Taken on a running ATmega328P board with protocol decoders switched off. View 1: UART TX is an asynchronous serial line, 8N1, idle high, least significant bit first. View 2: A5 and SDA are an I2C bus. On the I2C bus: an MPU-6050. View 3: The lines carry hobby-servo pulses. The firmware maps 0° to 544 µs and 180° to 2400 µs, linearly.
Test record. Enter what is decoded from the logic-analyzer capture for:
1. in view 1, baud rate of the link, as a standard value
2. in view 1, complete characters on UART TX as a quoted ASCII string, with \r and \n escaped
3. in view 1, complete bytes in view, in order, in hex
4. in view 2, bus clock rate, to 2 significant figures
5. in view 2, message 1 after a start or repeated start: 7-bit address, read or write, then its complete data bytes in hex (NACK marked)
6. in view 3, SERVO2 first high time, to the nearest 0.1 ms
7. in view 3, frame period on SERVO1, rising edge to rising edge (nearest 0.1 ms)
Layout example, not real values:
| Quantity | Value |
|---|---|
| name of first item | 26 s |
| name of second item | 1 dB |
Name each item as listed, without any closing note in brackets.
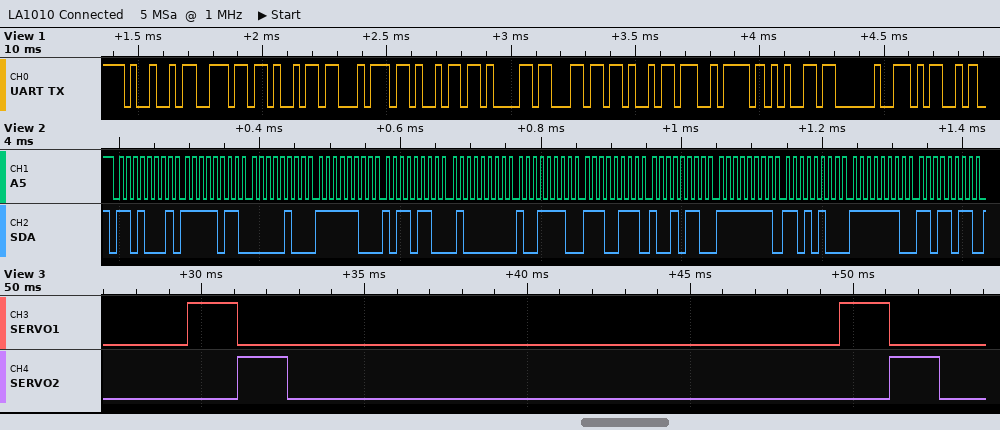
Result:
| Quantity | Value |
|---|---|
| in view 1, baud rate of the link, as a standard value | 38400 baud |
| in view 1, complete characters on UART TX as a quoted ASCII string, with \r and \n escaped | "Initialize M" |
| in view 1, complete bytes in view, in order, in hex | 49 6E 69 74 69 61 6C 69 7A 65 20 4D |
| in view 2, bus clock rate, to 2 significant figures | 100 kHz |
| in view 2, message 1 after a start or repeated start: 7-bit address, read or write, then its complete data bytes in hex | 0x68 read: FB 04 FC B6 40 9E E7 96 FF D4 FE DB |
| in view 3, SERVO2 first high time, to the nearest 0.1 ms | 1.5 ms |
| in view 3, frame period on SERVO1, rising edge to rising edge | 20.0 ms |
